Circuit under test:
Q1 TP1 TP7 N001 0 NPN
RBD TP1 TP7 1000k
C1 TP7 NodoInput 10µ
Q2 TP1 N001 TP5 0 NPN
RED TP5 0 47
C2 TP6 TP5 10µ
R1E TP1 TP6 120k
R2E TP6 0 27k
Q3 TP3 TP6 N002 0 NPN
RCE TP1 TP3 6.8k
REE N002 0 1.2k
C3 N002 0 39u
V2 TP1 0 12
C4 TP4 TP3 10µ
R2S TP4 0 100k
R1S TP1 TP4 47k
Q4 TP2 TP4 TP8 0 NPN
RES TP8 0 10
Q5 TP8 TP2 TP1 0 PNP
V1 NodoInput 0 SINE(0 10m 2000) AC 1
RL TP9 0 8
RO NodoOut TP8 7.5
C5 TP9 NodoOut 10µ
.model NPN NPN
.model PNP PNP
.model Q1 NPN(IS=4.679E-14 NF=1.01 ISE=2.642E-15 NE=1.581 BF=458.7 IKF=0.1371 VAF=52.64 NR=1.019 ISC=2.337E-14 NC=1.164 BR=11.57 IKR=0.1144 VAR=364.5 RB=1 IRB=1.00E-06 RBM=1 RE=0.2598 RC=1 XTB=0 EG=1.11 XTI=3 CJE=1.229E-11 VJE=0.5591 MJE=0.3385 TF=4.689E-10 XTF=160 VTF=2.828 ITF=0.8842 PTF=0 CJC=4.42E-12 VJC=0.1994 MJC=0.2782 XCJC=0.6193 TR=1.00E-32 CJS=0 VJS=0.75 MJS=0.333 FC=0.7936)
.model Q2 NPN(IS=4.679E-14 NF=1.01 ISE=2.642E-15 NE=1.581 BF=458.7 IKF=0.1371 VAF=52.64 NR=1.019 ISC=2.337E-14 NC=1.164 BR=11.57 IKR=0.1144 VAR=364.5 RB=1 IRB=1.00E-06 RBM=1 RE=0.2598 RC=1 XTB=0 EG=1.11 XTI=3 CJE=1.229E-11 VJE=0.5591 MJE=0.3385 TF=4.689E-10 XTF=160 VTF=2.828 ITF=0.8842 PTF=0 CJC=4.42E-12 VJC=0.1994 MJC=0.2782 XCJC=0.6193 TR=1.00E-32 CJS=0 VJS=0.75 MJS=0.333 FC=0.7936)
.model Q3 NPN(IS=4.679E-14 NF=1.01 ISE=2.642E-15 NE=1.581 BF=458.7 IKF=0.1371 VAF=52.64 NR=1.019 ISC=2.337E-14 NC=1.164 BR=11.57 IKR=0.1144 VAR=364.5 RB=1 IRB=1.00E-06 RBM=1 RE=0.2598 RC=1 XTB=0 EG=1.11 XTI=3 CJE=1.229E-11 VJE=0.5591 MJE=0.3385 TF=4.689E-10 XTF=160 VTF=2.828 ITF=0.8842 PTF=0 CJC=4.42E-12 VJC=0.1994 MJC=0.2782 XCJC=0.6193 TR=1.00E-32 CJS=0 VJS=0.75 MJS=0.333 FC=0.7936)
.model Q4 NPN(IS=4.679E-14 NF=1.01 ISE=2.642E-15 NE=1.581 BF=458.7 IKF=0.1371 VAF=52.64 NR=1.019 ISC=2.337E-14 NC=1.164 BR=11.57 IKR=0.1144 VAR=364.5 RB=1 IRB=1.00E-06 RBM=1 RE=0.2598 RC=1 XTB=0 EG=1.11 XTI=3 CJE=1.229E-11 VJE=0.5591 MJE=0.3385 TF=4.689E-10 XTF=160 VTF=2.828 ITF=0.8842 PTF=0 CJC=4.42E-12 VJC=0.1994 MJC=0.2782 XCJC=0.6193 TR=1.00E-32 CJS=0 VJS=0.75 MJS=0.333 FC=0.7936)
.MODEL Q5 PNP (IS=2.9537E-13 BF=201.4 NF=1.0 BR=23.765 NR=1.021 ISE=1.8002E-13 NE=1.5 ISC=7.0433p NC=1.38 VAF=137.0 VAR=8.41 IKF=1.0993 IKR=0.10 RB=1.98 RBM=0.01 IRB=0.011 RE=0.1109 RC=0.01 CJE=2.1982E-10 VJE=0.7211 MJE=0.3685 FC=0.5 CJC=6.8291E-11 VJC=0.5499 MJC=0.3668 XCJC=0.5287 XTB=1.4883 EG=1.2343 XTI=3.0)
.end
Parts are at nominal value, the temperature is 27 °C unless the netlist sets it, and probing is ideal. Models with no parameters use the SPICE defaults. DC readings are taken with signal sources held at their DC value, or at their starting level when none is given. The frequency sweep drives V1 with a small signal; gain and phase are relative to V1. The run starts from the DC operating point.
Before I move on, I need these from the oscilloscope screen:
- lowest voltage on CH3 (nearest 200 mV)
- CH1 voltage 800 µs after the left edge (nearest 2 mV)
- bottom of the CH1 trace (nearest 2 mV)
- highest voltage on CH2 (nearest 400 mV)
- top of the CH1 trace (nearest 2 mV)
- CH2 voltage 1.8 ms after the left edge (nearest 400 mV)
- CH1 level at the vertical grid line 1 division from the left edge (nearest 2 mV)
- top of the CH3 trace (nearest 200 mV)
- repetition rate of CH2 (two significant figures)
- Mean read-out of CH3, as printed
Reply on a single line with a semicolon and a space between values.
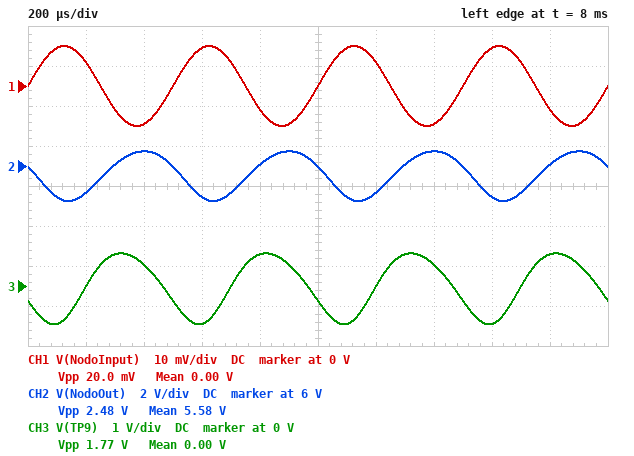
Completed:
-1.0 V; -6 mV; -10 mV; 6.8 V; 10 mV; 6.0 V; 6 mV; 800 mV; 2.0 kHz; 0.00 V
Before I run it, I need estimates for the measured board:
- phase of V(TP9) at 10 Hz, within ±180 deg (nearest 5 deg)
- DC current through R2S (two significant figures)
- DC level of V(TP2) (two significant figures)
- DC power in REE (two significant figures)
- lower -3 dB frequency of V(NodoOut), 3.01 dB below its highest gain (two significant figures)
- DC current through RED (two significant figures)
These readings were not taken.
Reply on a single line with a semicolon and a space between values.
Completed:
-15 deg; 64 µA; 11 V; 1.2 mW; 130 Hz; 71 mA
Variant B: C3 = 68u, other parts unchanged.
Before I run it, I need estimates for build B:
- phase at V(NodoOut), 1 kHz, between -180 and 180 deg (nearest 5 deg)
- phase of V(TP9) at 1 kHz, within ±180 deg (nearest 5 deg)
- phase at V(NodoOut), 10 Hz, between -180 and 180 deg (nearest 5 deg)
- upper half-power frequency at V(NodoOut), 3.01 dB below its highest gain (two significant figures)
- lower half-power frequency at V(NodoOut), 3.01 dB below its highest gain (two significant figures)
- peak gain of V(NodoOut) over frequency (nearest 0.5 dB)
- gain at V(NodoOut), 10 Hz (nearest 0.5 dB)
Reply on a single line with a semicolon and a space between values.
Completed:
165 deg; -130 deg; -100 deg; 1.8 kHz; 86 Hz; 45.5 dB; 26.0 dB
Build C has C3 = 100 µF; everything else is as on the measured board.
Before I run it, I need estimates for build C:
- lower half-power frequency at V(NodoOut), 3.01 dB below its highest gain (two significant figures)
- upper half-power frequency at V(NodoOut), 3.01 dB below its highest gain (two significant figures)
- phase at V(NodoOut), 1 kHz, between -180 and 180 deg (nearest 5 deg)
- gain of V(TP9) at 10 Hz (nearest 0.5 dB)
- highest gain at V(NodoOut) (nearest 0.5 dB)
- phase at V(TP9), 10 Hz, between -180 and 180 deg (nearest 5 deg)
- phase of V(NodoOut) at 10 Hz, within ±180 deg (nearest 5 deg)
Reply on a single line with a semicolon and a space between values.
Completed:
62 Hz; 1.7 kHz; 165 deg; -17.0 dB; 45.5 dB; -10 deg; -100 deg
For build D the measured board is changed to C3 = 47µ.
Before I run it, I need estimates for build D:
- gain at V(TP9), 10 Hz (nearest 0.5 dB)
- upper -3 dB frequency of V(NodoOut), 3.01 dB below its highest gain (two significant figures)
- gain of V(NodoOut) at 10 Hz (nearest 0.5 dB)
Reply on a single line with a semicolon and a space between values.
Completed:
-22.5 dB; 2.0 kHz; 23.5 dB
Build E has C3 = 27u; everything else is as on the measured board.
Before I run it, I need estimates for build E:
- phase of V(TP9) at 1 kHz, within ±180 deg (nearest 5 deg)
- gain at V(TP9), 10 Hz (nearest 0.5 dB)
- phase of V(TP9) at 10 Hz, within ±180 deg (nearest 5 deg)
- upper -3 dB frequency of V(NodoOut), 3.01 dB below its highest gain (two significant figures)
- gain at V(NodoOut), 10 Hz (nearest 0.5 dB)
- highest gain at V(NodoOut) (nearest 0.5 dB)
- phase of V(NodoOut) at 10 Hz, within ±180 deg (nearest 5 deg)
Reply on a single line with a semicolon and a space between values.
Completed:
-120 deg; -26.5 dB; -20 deg; 2.5 kHz; 19.5 dB; 44.5 dB; -110 deg
